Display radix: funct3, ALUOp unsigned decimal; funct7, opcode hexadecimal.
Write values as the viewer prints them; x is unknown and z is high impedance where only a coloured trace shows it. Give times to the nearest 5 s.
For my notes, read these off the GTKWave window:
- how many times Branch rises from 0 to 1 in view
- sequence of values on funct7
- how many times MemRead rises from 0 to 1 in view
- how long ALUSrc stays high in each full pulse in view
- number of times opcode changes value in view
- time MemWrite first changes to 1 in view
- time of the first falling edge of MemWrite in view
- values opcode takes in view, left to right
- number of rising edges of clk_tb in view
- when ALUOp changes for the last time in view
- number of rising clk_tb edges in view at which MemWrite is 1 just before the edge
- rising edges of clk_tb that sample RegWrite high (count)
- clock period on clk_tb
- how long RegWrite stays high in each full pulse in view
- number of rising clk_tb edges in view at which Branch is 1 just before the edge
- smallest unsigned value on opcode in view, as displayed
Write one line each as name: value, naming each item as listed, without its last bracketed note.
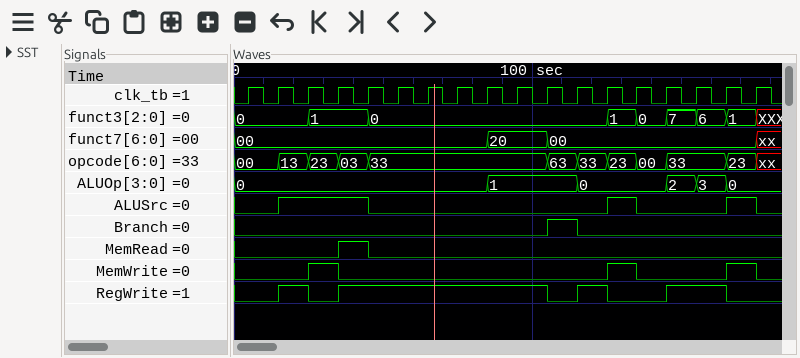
how many times Branch rises from 0 to 1 in view: 1
sequence of values on funct7: 00, 20, 00, xx
how many times MemRead rises from 0 to 1 in view: 1
how long ALUSrc stays high in each full pulse in view: 30 s, 10 s, 10 s
number of times opcode changes value in view: 11
time MemWrite first changes to 1 in view: 25 s
time of the first falling edge of MemWrite in view: 35 s
values opcode takes in view, left to right: 00, 13, 23, 03, 33, 63, 33, 23, 00, 33, 23, xx
number of rising edges of clk_tb in view: 18
when ALUOp changes for the last time in view: 165 s
number of rising clk_tb edges in view at which MemWrite is 1 just before the edge: 3
rising edges of clk_tb that sample RegWrite high: 11
clock period on clk_tb: 10 s
how long RegWrite stays high in each full pulse in view: 10 s, 70 s, 10 s, 20 s
number of rising clk_tb edges in view at which Branch is 1 just before the edge: 1
smallest unsigned value on opcode in view, as displayed: 00
